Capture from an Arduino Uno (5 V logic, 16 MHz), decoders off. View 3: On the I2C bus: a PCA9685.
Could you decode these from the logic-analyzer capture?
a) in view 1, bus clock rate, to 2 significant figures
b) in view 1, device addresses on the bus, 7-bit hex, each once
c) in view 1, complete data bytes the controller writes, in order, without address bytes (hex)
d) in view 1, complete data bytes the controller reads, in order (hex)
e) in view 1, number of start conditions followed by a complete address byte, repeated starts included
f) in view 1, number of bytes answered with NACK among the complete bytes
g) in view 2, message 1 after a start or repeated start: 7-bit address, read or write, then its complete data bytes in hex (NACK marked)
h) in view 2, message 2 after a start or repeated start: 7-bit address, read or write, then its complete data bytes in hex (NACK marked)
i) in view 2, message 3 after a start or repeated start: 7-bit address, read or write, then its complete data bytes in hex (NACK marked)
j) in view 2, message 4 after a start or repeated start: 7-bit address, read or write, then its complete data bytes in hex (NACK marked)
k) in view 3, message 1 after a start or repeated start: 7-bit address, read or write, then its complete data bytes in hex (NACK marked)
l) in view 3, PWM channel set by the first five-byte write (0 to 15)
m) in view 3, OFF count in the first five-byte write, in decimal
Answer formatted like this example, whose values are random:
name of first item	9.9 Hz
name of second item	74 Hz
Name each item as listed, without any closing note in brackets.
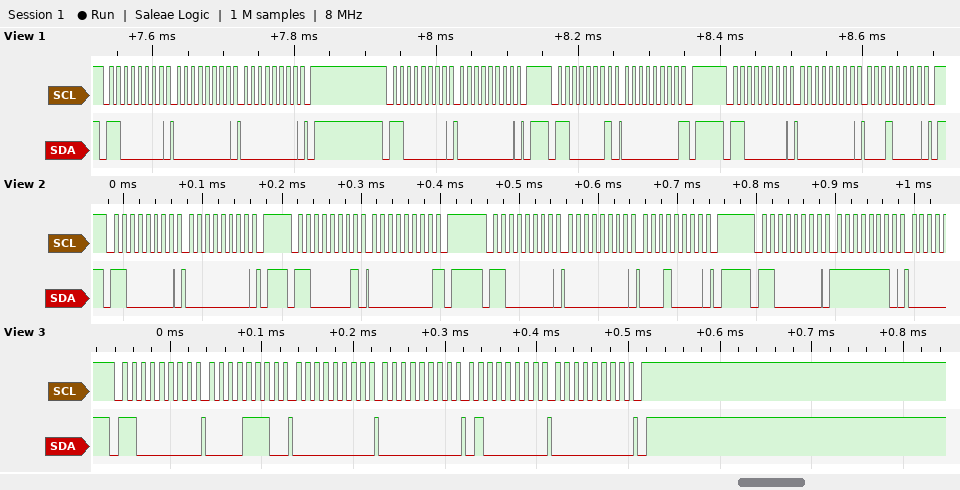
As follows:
in view 1, bus clock rate, to 2 significant figures	100 kHz
in view 1, device addresses on the bus, 7-bit hex, each once	0x60
in view 1, complete data bytes the controller writes, in order, without address bytes	00 00 00 00 10
in view 1, complete data bytes the controller reads, in order	00
in view 1, number of start conditions followed by a complete address byte, repeated starts included	4
in view 1, number of bytes answered with NACK among the complete bytes	1
in view 2, message 1 after a start or repeated start: 7-bit address, read or write, then its complete data bytes in hex	0x60 write: 00
in view 2, message 2 after a start or repeated start: 7-bit address, read or write, then its complete data bytes in hex	0x60 read: 00 NACK
in view 2, message 3 after a start or repeated start: 7-bit address, read or write, then its complete data bytes in hex	0x60 write: 00 10
in view 2, message 4 after a start or repeated start: 7-bit address, read or write, then its complete data bytes in hex	0x60 write: FE
in view 3, message 1 after a start or repeated start: 7-bit address, read or write, then its complete data bytes in hex	0x60 write: 0E 00 00 40 00
in view 3, PWM channel set by the first five-byte write	2
in view 3, OFF count in the first five-byte write, in decimal	64
